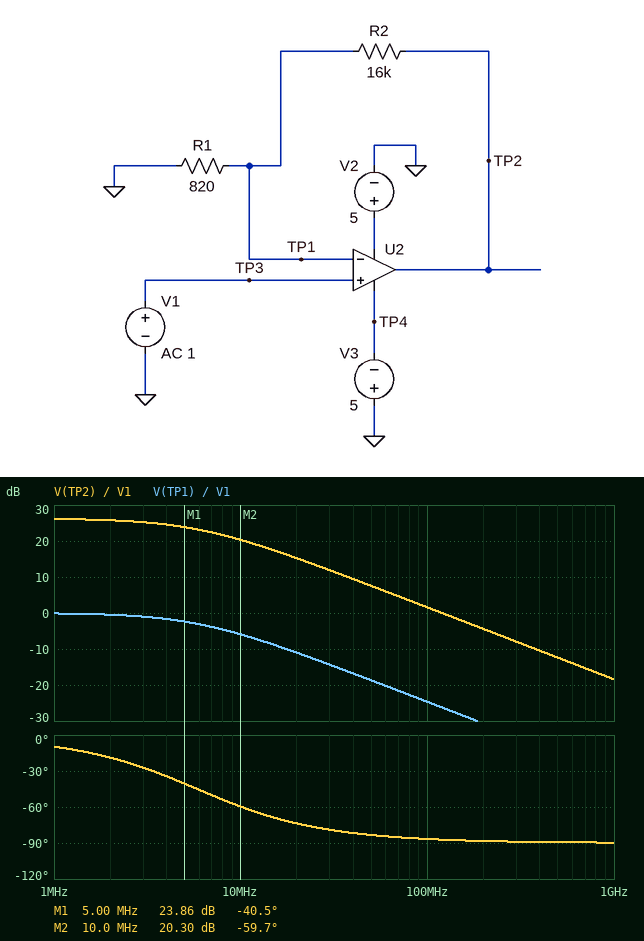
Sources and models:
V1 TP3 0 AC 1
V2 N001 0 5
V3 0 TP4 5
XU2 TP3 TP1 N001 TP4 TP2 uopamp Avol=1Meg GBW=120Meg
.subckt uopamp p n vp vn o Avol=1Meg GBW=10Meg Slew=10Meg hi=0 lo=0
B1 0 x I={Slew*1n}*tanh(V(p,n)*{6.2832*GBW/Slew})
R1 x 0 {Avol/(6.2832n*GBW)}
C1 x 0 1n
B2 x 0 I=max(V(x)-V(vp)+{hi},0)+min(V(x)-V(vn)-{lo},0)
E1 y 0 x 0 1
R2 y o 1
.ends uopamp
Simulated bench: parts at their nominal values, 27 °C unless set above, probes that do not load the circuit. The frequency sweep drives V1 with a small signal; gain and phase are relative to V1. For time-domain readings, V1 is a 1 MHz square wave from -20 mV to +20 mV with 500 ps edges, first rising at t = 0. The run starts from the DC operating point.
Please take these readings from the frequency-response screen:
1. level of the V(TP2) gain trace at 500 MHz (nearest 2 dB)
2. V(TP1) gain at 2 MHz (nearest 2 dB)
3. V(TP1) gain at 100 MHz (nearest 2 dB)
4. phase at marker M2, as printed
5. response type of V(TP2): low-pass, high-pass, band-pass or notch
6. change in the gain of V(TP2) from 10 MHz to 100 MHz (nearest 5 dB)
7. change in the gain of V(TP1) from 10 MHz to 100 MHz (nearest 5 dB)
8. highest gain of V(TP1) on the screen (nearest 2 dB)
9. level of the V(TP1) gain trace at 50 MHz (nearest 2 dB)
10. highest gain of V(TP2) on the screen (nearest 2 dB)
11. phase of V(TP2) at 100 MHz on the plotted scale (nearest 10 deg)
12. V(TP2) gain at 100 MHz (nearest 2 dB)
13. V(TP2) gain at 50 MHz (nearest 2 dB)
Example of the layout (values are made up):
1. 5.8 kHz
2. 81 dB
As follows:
1. -12 dB
2. 0 dB
3. -24 dB
4. -59.7 deg
5. low-pass
6. -20 dB
7. -20 dB
8. 0 dB
9. -18 dB
10. 26 dB
11. -90 deg
12. 2 dB
13. 8 dB
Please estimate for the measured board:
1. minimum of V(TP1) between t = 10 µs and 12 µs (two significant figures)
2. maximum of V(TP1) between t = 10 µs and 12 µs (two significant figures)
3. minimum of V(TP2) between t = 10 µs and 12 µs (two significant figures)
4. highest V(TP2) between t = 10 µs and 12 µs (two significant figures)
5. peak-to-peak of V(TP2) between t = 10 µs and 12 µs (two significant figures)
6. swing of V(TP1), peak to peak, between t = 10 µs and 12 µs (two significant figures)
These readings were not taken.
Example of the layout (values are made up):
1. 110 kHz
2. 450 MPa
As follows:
1. -20 mV
2. 20 mV
3. -410 mV
4. 410 mV
5. 820 mV
6. 40 mV
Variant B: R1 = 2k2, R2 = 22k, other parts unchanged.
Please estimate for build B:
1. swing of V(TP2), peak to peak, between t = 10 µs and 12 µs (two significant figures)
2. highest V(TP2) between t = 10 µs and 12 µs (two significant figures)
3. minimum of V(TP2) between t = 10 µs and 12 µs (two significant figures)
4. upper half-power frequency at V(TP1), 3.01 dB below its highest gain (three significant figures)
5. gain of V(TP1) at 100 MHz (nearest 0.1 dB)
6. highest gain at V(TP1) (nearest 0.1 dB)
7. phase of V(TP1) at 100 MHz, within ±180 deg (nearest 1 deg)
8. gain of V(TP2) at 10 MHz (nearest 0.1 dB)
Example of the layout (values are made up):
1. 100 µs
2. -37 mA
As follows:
1. 440 mV
2. 220 mV
3. -220 mV
4. 10.9 MHz
5. -19.3 dB
6. 0 dB
7. -84 deg
8. 18.2 dB
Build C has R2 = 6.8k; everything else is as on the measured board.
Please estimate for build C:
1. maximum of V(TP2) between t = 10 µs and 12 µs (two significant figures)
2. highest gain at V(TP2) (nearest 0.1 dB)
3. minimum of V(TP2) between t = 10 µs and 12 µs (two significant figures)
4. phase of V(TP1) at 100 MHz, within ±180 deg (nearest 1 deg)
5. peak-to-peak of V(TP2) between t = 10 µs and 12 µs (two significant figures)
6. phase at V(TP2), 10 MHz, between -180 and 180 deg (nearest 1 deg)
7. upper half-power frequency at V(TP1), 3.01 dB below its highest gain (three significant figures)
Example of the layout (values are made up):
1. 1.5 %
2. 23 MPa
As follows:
1. 190 mV
2. 19.4 dB
3. -190 mV
4. -83 deg
5. 370 mV
6. -38 deg
7. 12.9 MHz
